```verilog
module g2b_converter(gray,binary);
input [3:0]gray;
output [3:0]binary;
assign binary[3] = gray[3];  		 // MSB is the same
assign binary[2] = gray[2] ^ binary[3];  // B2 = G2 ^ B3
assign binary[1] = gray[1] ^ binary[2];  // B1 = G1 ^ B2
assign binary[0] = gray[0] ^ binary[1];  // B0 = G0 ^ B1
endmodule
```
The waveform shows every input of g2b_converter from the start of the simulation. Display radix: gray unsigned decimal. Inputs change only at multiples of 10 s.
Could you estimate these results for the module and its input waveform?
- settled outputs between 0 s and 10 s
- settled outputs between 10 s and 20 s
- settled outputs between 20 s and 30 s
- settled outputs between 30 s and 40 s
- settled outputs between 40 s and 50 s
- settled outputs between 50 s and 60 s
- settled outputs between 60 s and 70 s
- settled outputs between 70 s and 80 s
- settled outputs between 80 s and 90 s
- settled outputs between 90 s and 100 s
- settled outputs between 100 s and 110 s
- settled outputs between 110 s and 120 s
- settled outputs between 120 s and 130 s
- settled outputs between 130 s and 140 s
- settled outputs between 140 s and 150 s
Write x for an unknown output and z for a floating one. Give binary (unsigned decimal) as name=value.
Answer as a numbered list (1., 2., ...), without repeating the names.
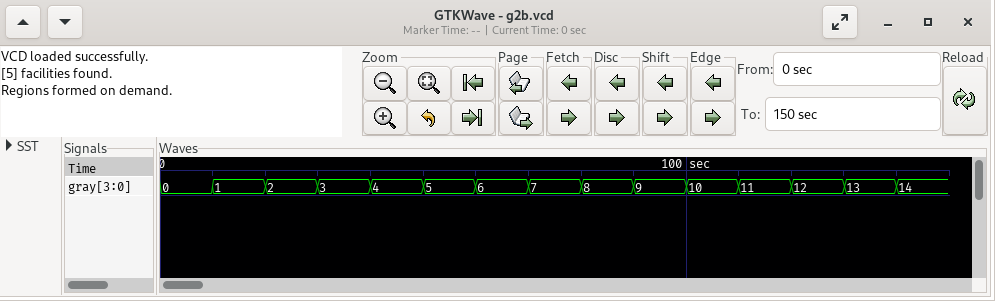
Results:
1. binary=0
2. binary=1
3. binary=3
4. binary=2
5. binary=7
6. binary=6
7. binary=4
8. binary=5
9. binary=15
10. binary=14
11. binary=12
12. binary=13
13. binary=8
14. binary=9
15. binary=11
